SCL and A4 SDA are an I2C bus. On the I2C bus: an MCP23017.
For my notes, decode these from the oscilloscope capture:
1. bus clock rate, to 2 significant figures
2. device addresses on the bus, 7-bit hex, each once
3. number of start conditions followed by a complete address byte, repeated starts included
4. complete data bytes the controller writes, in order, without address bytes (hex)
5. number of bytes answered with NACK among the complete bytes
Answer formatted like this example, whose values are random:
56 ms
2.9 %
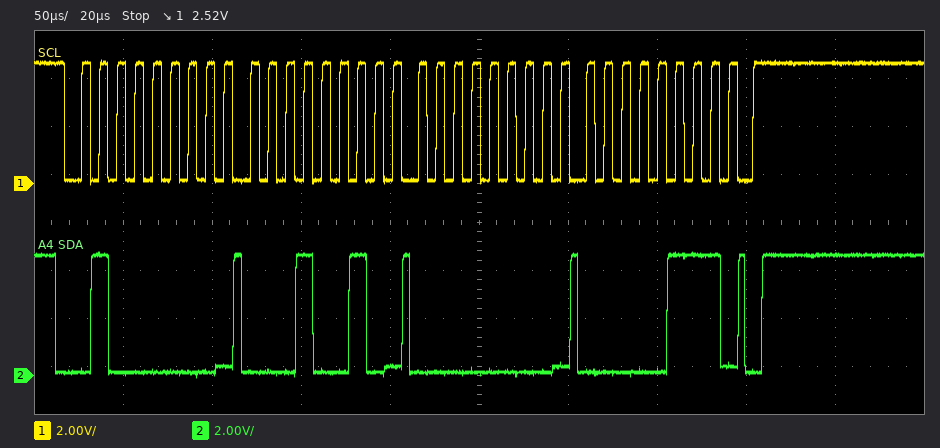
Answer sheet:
100 kHz
0x20
1
12 00 07
0
